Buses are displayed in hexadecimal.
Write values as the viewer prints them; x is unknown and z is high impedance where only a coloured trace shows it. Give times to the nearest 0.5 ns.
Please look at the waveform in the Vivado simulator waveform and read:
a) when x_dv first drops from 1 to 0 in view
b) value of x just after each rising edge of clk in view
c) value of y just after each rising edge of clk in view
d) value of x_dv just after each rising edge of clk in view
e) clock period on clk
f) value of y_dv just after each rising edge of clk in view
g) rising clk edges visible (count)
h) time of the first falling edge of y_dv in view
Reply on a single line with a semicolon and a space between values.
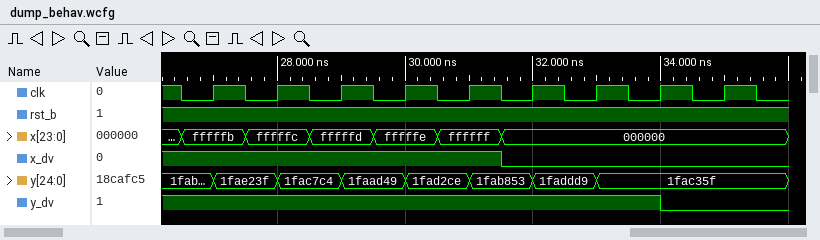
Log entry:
31.5 ns; fffffb, fffffc, fffffd, fffffe, ffffff, 000000, 000000, 000000, 000000; 1fae23f, 1fac7c4, 1faad49, 1fad2ce, 1fab853, 1faddd9, 1fac35f, 1fac35f, 1fac35f; 1 1 1 1 1 0 0 0 0; 1 ns; 1 1 1 1 1 1 1 0 0; 9; 34 ns
